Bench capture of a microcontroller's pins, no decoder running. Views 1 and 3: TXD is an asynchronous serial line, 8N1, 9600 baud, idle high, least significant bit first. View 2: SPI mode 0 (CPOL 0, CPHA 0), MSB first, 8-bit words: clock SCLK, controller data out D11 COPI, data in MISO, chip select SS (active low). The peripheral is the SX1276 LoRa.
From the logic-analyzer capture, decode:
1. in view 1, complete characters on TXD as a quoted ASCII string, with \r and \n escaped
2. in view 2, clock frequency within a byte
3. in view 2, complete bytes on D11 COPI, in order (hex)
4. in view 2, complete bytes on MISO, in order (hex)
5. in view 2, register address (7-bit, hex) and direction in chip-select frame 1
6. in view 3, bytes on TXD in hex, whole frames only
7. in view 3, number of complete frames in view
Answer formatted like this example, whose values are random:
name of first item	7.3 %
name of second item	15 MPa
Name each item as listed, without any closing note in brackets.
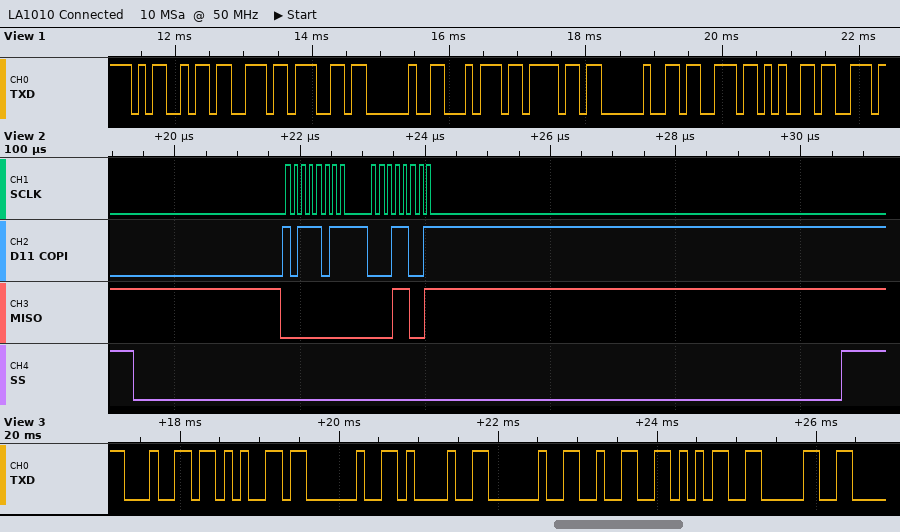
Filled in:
in view 1, complete characters on TXD as a quoted ASCII string, with \r and \n escaped	"Msg to se"
in view 2, clock frequency within a byte	8 MHz
in view 2, complete bytes on D11 COPI, in order	BB 19
in view 2, complete bytes on MISO, in order	00 19
in view 2, register address (7-bit, hex) and direction in chip-select frame 1	0x3B write
in view 3, bytes on TXD in hex, whole frames only	64 65 20 21 20 32 35 30
in view 3, number of complete frames in view	8
